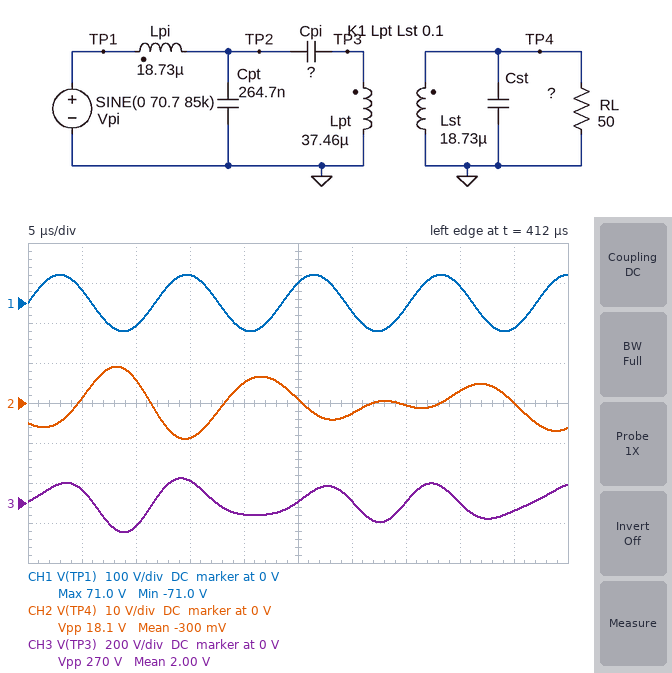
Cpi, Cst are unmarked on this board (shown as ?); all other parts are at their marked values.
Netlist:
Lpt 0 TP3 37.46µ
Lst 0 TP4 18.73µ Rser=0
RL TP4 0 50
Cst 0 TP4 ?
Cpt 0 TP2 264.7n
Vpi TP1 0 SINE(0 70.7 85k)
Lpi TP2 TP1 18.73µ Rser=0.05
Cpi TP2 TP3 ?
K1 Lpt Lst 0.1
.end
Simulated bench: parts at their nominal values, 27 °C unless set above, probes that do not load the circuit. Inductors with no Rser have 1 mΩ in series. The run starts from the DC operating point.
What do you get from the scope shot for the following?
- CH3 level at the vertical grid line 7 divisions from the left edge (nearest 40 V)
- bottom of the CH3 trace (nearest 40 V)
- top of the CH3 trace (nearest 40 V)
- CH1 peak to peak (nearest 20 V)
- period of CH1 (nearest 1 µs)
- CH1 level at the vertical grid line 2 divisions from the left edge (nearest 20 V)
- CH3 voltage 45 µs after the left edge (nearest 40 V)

0 V
-160 V
120 V
140 V
12 µs
-60 V
-40 V
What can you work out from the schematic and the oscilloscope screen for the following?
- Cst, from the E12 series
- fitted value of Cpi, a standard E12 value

470 nF
56 nF
